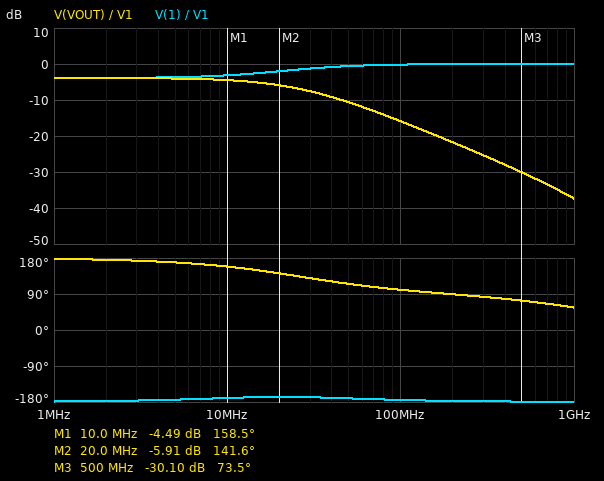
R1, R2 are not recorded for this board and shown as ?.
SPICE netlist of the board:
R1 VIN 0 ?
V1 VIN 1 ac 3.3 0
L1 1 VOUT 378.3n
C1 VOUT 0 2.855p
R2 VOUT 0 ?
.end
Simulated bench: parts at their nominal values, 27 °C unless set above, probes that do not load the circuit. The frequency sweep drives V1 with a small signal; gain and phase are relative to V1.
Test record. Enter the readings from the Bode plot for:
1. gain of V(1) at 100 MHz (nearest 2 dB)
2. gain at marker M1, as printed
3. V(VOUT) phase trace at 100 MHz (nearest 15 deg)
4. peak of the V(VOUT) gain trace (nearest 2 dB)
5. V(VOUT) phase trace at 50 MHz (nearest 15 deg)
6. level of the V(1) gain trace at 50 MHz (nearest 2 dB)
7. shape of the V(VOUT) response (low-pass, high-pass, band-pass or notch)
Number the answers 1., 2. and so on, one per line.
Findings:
1. 0 dB
2. -4.49 dB
3. 105 deg
4. -4 dB
5. 120 deg
6. 0 dB
7. low-pass
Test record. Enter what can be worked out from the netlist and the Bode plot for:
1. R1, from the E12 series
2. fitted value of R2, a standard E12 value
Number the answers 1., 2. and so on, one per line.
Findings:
1. 22 Ω
2. 39 Ω
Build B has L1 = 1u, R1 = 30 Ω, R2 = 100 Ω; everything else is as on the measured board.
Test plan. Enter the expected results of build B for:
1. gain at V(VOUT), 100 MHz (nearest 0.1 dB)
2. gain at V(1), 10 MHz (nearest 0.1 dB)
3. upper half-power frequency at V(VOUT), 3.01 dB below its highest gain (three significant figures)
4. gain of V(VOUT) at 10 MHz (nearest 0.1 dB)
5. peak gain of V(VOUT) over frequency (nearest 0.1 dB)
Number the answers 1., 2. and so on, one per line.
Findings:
1. -16.0 dB
2. -1.8 dB
3. 21.3 MHz
4. -3.1 dB
5. -2.3 dB
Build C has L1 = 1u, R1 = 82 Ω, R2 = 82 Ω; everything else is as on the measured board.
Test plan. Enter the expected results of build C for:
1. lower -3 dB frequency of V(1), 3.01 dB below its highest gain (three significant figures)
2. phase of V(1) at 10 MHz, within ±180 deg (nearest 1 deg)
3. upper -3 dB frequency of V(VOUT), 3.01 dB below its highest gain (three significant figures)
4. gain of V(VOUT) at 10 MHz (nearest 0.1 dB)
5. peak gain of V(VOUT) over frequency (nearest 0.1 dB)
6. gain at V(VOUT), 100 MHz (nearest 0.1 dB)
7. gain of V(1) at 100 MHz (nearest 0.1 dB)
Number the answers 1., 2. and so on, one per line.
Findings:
1. 18.8 MHz
2. -164 deg
3. 26.6 MHz
4. -6.6 dB
5. -6.0 dB
6. -17.9 dB
7. -0.2 dB
